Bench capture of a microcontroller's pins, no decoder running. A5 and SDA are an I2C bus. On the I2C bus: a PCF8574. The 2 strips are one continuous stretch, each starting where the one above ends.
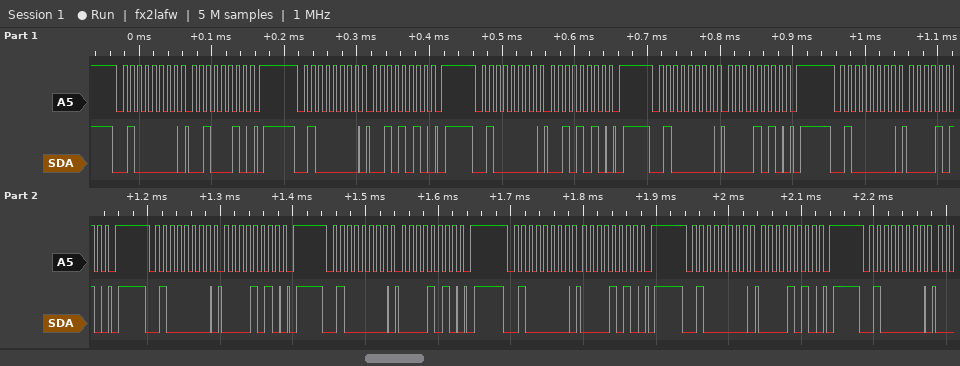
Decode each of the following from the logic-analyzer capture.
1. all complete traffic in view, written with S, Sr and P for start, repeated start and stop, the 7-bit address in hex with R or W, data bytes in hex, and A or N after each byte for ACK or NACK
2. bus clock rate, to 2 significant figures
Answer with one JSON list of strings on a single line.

["S 20W A 22 A P S 20W A 2A A P S 20W A 2A A P S 20W A 0A A P S 20W A 0A A P S 20W A 0A A P S 20W A 0A A P S 20W A 0A A P S 20W A 0A A P S 20W A", "100 kHz"]
